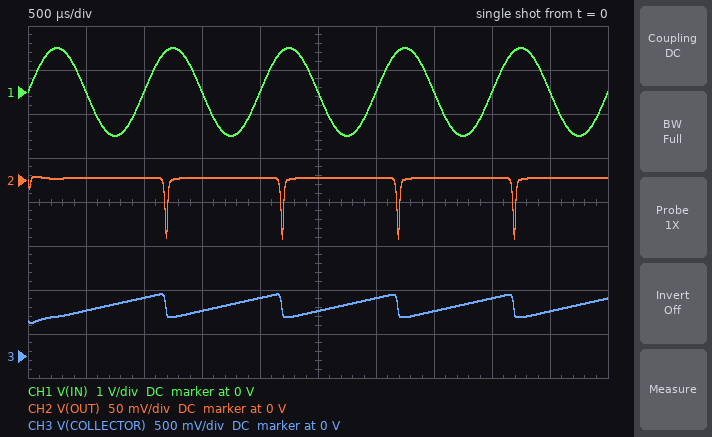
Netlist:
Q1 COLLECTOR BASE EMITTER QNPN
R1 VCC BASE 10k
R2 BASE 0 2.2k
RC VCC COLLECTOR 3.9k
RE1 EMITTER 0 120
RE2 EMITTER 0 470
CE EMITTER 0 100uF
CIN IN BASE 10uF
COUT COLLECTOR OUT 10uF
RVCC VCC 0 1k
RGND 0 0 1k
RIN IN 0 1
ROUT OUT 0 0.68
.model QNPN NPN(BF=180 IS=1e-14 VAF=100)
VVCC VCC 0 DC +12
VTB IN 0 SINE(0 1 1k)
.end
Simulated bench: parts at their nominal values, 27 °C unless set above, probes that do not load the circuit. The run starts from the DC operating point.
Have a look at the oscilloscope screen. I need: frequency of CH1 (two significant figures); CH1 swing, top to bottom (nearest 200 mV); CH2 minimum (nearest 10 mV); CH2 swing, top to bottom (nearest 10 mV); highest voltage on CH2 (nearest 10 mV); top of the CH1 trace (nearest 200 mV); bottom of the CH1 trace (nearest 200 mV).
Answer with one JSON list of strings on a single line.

["1.0 kHz", "2.0 V", "-70 mV", "70 mV", "0 V", "1.0 V", "-1.0 V"]
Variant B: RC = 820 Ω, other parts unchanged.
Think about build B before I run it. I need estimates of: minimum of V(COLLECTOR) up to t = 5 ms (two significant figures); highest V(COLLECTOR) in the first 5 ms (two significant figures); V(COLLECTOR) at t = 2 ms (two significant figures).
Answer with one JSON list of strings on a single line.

["1.3 V", "2.4 V", "2.3 V"]
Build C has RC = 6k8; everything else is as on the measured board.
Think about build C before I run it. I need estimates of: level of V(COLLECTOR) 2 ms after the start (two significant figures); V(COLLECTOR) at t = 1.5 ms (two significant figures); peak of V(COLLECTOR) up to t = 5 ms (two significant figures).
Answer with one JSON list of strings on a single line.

["450 mV", "370 mV", "480 mV"]
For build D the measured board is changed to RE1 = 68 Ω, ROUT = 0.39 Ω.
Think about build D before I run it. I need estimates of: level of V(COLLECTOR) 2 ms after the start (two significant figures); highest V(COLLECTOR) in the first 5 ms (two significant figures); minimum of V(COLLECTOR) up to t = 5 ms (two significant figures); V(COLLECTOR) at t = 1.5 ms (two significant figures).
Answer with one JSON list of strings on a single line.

["530 mV", "580 mV", "250 mV", "380 mV"]
